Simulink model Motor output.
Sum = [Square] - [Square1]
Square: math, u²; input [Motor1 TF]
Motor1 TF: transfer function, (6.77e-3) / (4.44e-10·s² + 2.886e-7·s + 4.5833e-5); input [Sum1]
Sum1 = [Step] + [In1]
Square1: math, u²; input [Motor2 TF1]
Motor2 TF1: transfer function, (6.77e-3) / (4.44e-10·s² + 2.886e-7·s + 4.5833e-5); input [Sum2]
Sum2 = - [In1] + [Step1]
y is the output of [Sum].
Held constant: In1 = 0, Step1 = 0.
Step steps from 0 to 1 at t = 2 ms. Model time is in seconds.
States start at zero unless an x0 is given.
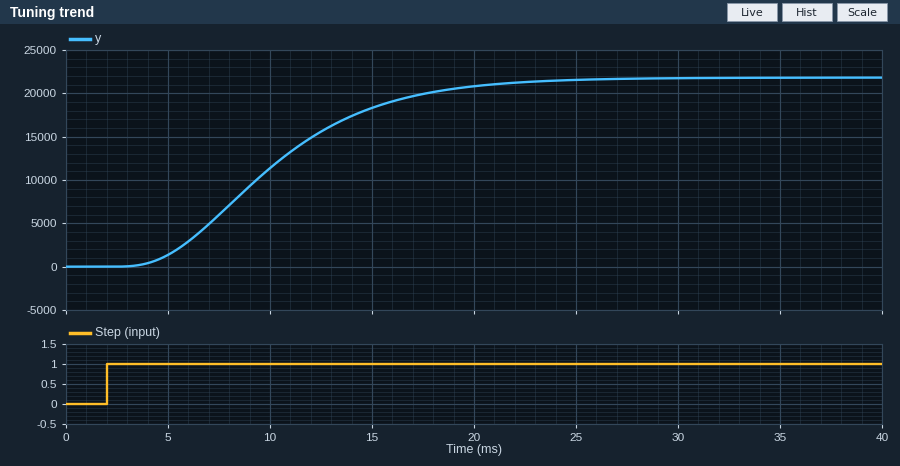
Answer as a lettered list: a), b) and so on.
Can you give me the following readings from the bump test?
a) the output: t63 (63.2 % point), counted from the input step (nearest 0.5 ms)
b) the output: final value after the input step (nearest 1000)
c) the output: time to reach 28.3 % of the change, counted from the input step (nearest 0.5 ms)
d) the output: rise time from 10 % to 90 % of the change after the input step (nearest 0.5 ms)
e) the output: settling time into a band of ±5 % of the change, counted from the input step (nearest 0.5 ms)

a) 9.5 ms
b) 22000
c) 5.5 ms
d) 11.5 ms
e) 17.5 ms
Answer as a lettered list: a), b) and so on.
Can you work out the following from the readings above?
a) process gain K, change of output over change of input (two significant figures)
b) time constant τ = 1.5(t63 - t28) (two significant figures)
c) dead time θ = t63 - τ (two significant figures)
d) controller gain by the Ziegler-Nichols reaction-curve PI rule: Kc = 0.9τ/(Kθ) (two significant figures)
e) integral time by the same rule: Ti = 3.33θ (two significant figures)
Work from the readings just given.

a) 22000
b) 6.0 ms
c) 3.5 ms
d) 0.000070
e) 12 ms
